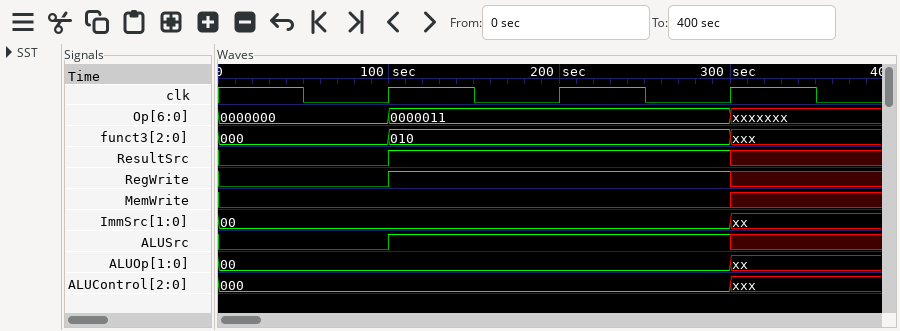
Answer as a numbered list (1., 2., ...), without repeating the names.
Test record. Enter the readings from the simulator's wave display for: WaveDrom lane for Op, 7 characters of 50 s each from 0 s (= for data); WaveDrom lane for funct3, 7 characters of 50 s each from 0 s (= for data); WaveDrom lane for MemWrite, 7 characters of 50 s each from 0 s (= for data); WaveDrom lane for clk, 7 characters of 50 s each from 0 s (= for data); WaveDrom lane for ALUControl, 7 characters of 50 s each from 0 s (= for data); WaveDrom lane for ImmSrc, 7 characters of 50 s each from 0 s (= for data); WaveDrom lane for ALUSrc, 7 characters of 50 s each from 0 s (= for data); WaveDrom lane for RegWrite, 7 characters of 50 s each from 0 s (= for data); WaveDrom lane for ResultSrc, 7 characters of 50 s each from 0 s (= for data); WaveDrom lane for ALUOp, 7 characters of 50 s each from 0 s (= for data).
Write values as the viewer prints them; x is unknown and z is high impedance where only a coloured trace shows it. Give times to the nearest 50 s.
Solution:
1. {name: 'Op', wave: '=.=...x', data: '0000000 0000011'}
2. {name: 'funct3', wave: '=.=...x', data: '000 010'}
3. {name: 'MemWrite', wave: '0.....x'}
4. {name: 'clk', wave: '1010101'}
5. {name: 'ALUControl', wave: '=.....x', data: '000'}
6. {name: 'ImmSrc', wave: '=.....x', data: '00'}
7. {name: 'ALUSrc', wave: '0.1...x'}
8. {name: 'RegWrite', wave: '0.1...x'}
9. {name: 'ResultSrc', wave: '0.1...x'}
10. {name: 'ALUOp', wave: '=.....x', data: '00'}
